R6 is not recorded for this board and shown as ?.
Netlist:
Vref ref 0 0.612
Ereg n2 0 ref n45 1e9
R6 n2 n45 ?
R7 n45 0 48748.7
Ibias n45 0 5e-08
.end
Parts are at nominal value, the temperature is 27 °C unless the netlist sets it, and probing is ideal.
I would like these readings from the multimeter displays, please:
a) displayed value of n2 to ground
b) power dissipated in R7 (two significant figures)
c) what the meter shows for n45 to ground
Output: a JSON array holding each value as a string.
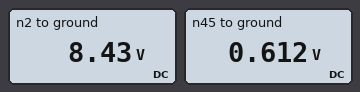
["8.43 V", "7.7 µW", "0.612 V"]
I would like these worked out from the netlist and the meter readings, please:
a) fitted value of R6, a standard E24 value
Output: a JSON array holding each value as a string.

["620 kΩ"]
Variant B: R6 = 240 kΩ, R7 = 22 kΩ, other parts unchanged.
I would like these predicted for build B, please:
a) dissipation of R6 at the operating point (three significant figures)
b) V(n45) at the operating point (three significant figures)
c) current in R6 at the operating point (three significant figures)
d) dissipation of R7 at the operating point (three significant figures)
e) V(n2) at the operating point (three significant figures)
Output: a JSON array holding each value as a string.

["186 µW", "612 mV", "27.9 µA", "17.0 µW", "7.30 V"]
